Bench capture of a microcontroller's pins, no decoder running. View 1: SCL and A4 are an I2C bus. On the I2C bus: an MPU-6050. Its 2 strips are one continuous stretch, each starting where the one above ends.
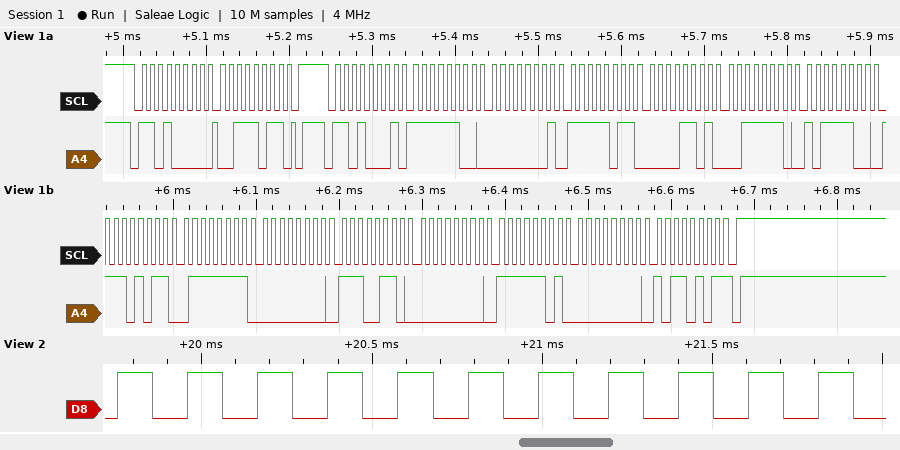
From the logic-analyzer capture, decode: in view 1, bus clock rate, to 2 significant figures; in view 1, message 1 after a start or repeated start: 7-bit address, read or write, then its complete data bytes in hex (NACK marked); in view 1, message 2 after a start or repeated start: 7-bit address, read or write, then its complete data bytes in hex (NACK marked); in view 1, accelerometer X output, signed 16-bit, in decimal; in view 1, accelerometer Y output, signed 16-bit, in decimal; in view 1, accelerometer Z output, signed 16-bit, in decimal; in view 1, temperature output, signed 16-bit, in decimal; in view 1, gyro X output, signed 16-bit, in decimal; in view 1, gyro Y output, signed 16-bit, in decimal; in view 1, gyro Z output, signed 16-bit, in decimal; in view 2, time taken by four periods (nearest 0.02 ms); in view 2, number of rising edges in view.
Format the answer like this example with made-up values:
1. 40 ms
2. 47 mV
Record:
1. 100 kHz
2. 0x68 write: 3B
3. 0x68 read: FC 01 FB 0D 3E BC EB 7F 00 E6 00 FD 00 B5 NACK
4. -1023
5. -1267
6. 16060
7. -5249
8. 230
9. 253
10. 181
11. 0.82 ms
12. 11
